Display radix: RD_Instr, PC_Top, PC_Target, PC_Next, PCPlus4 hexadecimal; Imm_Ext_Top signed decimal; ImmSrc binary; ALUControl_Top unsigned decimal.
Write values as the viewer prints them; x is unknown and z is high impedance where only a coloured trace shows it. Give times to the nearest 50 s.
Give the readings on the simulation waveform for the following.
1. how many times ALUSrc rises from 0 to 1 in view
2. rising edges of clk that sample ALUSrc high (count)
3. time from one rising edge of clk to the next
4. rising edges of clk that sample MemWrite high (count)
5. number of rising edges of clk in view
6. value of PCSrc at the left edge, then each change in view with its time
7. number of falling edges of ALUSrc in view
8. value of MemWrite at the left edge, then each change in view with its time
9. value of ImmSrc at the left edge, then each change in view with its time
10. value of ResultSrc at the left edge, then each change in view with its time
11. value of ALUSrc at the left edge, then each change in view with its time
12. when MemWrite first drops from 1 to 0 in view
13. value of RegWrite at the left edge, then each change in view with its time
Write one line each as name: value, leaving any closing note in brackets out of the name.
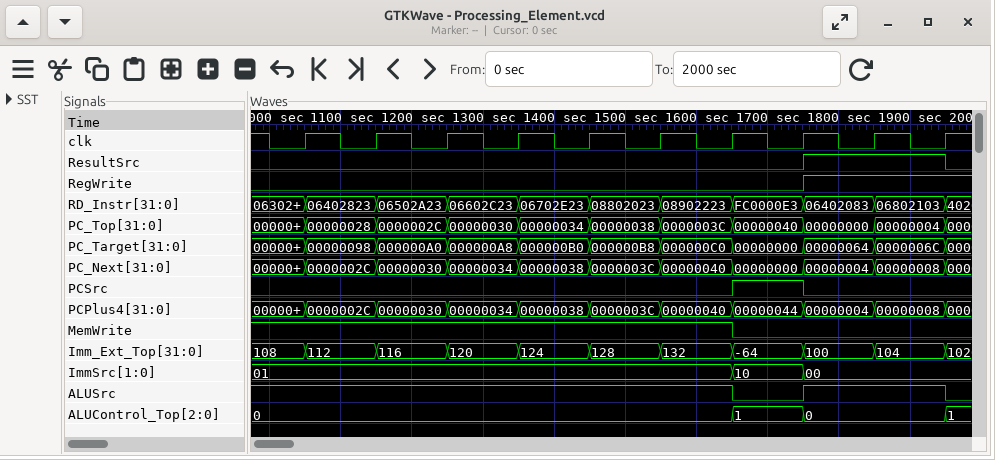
how many times ALUSrc rises from 0 to 1 in view: 1
rising edges of clk that sample ALUSrc high: 9
time from one rising edge of clk to the next: 100 s
rising edges of clk that sample MemWrite high: 7
number of rising edges of clk in view: 10
value of PCSrc at the left edge, then each change in view with its time: 0, 1 at 1650 s, 0 at 1750 s
number of falling edges of ALUSrc in view: 2
value of MemWrite at the left edge, then each change in view with its time: 1, 0 at 1650 s
value of ImmSrc at the left edge, then each change in view with its time: 01, 10 at 1650 s, 00 at 1750 s
value of ResultSrc at the left edge, then each change in view with its time: 0, 1 at 1750 s, 0 at 1950 s
value of ALUSrc at the left edge, then each change in view with its time: 1, 0 at 1650 s, 1 at 1750 s, 0 at 1950 s
when MemWrite first drops from 1 to 0 in view: 1650 s
value of RegWrite at the left edge, then each change in view with its time: 0, 1 at 1750 s
